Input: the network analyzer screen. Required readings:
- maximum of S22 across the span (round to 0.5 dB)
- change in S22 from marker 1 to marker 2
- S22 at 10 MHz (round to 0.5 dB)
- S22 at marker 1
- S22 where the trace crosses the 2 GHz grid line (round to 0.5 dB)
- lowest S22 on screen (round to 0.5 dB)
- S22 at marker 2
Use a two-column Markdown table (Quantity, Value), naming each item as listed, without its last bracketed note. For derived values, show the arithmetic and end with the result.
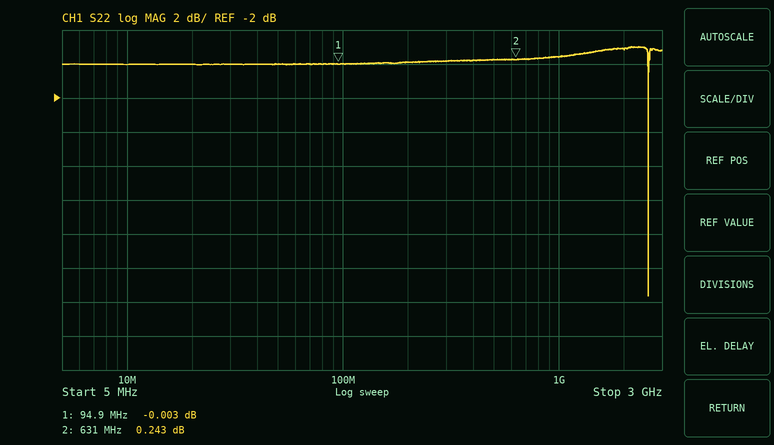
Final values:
| Quantity | Value |
|---|---|
| maximum of S22 across the span | 1.0 dB |
| change in S22 from marker 1 to marker 2 | 0.243 − (-0.003) = 0.246 dB |
| S22 at 10 MHz | 0.0 dB |
| S22 at marker 1 | -0.003 dB |
| S22 where the trace crosses the 2 GHz grid line | 1.0 dB |
| lowest S22 on screen | -13.5 dB |
| S22 at marker 2 | 0.243 dB |
